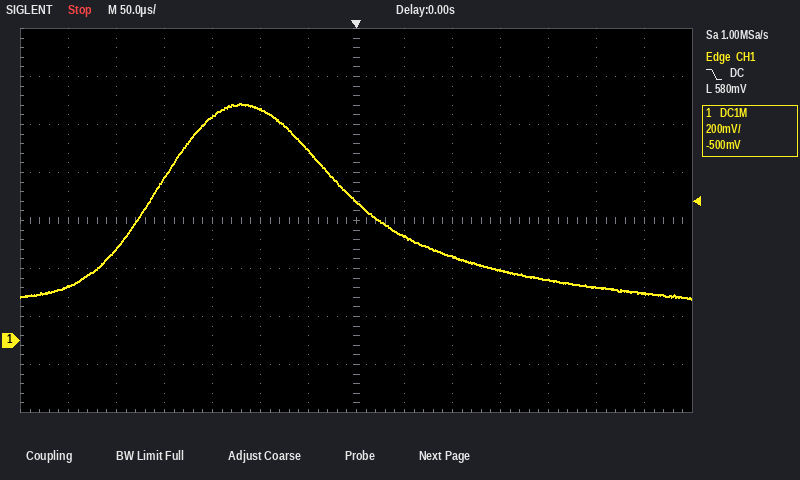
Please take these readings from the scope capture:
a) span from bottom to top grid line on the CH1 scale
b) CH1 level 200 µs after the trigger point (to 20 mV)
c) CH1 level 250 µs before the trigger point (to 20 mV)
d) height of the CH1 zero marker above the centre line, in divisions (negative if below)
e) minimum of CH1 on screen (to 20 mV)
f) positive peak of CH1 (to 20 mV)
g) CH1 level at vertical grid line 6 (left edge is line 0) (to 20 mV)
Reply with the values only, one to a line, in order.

1.6 V
260 mV
380 mV
-2.5 div
180 mV
980 mV
800 mV
